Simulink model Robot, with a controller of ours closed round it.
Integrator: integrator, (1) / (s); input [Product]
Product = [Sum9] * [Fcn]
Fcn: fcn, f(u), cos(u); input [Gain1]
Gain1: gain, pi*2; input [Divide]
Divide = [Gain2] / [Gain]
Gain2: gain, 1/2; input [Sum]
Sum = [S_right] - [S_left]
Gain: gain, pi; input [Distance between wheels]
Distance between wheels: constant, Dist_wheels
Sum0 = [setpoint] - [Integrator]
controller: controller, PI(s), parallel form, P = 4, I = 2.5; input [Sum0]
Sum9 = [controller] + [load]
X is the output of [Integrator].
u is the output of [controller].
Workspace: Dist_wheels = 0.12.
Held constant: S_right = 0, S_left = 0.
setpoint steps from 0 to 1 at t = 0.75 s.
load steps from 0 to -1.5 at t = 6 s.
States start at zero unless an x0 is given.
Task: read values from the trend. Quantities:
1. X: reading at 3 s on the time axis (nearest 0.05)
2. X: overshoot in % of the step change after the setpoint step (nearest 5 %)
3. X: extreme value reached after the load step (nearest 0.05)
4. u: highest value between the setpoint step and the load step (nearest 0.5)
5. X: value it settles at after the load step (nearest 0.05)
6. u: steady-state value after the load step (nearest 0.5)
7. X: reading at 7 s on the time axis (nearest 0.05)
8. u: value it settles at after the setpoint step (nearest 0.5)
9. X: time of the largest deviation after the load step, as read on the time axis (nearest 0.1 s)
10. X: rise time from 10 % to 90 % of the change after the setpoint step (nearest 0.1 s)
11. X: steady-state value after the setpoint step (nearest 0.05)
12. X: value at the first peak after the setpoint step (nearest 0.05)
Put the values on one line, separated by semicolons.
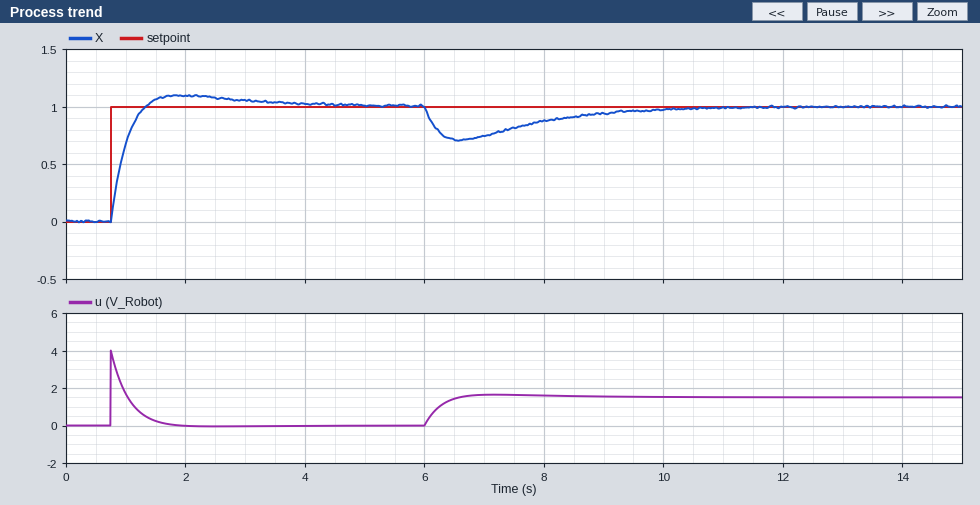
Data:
1.05; 10 %; 0.70; 4.0; 1.00; 1.5; 0.75; 0.0; 6.6 s; 0.4 s; 1.00; 1.10
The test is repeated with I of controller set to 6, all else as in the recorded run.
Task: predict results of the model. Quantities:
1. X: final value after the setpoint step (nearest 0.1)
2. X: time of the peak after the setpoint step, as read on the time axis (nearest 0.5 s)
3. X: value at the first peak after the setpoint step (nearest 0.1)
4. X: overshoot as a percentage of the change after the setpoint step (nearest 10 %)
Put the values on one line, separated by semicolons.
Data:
1.0; 1.5 s; 1.2; 20 %
